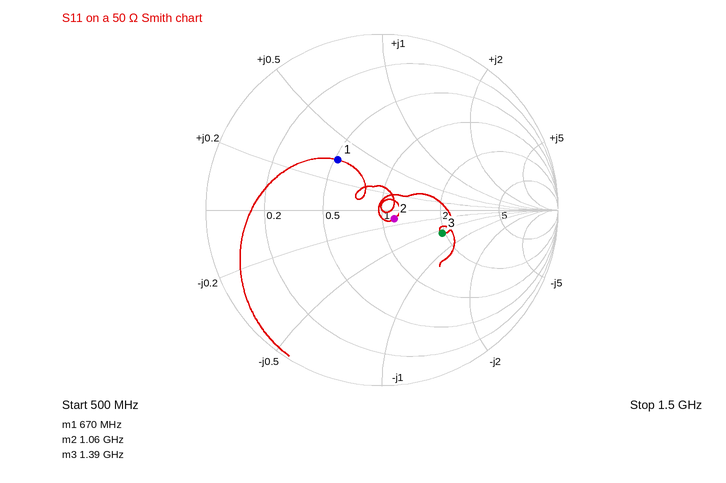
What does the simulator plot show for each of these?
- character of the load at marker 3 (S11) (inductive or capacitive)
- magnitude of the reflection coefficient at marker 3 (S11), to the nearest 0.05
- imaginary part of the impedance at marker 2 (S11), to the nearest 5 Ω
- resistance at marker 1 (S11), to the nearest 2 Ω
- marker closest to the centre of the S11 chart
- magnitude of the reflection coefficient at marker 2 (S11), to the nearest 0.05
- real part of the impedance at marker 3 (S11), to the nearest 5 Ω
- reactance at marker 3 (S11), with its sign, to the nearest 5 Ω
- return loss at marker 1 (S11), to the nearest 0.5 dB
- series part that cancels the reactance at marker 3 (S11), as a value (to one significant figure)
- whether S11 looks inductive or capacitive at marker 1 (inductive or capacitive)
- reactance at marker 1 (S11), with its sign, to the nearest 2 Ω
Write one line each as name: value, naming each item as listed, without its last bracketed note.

character of the load at marker 3 (S11): capacitive
magnitude of the reflection coefficient at marker 3 (S11), to the nearest 0.05: 0.35
imaginary part of the impedance at marker 2 (S11), to the nearest 5 Ω: -5 Ω
resistance at marker 1 (S11), to the nearest 2 Ω: 26 Ω
marker closest to the centre of the S11 chart: marker 2
magnitude of the reflection coefficient at marker 2 (S11), to the nearest 0.05: 0.10
real part of the impedance at marker 3 (S11), to the nearest 5 Ω: 95 Ω
reactance at marker 3 (S11), with its sign, to the nearest 5 Ω: -30 Ω
return loss at marker 1 (S11), to the nearest 0.5 dB: 8.5 dB
series part that cancels the reactance at marker 3 (S11), as a value: 3 nH
whether S11 looks inductive or capacitive at marker 1: inductive
reactance at marker 1 (S11), with its sign, to the nearest 2 Ω: +18 Ω
